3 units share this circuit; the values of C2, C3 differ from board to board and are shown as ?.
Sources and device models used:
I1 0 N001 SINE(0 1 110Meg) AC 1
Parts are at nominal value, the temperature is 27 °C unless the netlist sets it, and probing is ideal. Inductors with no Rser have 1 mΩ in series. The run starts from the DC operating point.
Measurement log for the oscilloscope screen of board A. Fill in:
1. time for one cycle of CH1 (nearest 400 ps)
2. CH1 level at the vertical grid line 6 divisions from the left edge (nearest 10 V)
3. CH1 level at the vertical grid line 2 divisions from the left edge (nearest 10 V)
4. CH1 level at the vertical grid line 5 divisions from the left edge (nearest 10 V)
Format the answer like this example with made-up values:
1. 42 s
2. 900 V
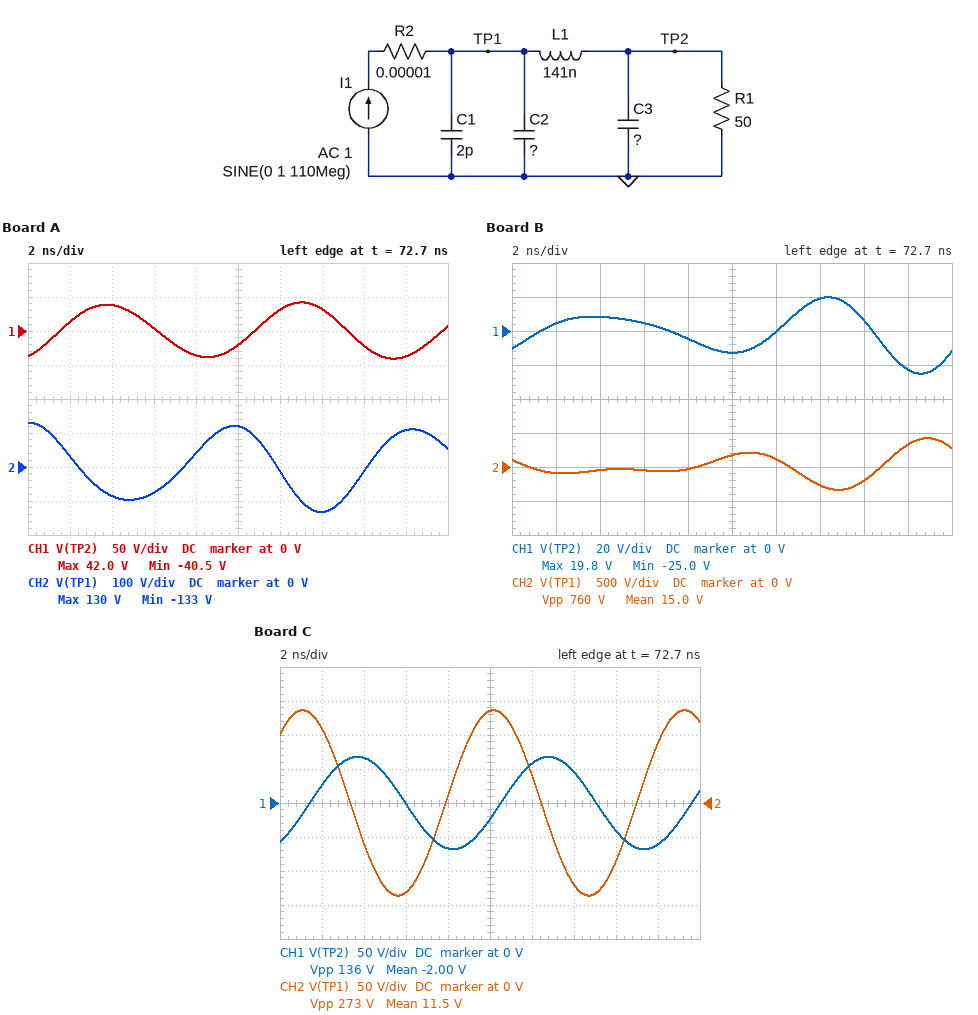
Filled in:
1. 9.2 ns
2. 30 V
3. 40 V
4. -20 V
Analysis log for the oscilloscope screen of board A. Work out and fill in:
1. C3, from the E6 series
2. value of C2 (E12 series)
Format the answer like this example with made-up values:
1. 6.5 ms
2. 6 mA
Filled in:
1. 47 pF
2. 4.7 pF
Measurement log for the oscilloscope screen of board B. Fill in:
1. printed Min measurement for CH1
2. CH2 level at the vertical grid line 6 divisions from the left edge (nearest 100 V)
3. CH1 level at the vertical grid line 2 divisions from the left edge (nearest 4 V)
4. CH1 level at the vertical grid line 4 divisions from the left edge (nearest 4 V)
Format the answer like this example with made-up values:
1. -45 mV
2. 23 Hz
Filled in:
1. -25.0 V
2. 100 V
3. 8 V
4. -4 V
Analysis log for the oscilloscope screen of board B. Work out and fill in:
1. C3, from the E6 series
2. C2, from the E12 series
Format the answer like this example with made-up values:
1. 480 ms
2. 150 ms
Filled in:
1. 220 pF
2. 8.2 pF
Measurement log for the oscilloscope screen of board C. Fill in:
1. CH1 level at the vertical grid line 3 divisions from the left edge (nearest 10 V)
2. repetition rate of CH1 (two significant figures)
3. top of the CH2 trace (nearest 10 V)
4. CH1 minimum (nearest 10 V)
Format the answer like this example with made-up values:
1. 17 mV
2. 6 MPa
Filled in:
1. 0 V
2. 110 MHz
3. 140 V
4. -70 V
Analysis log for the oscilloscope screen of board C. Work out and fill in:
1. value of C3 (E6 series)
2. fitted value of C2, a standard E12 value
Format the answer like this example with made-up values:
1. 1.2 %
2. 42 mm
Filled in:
1. 22 pF
2. 6.8 pF
